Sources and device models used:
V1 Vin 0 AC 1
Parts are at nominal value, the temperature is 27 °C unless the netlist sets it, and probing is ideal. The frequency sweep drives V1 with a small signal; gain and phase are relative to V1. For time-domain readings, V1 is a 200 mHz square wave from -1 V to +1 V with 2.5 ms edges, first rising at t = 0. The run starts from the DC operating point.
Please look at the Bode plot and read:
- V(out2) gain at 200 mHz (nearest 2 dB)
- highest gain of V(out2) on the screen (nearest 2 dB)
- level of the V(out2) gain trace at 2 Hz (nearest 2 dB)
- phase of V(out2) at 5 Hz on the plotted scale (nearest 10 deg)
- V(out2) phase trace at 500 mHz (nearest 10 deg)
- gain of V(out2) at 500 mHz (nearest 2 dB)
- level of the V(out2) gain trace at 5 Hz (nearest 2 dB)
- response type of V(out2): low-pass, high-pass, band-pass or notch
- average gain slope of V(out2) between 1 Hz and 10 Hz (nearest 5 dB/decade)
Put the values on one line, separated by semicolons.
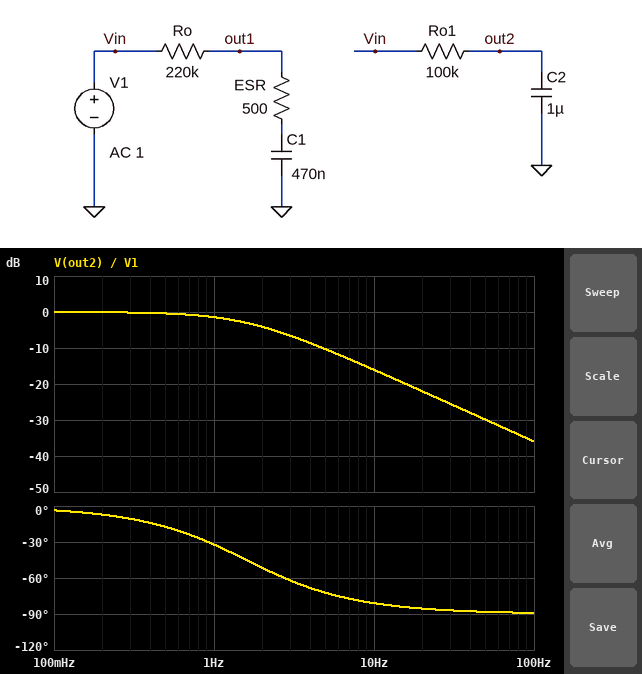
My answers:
0 dB; 0 dB; -4 dB; -70 deg; -20 deg; 0 dB; -10 dB; low-pass; -15 dB/decade
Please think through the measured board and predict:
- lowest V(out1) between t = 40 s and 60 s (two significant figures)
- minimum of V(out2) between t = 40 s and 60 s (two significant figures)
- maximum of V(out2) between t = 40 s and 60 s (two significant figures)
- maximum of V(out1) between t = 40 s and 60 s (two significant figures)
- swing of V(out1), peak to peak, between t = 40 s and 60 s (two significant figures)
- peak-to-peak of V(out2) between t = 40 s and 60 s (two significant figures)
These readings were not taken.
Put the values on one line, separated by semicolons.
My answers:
-1.0 V; -1.0 V; 1.0 V; 1.0 V; 2.0 V; 2.0 V
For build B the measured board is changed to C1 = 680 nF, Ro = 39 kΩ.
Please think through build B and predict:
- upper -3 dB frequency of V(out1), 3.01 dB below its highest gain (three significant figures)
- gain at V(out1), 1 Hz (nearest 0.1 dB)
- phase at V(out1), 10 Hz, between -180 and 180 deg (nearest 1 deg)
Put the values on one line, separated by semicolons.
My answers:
5.93 Hz; -0.1 dB; -58 deg
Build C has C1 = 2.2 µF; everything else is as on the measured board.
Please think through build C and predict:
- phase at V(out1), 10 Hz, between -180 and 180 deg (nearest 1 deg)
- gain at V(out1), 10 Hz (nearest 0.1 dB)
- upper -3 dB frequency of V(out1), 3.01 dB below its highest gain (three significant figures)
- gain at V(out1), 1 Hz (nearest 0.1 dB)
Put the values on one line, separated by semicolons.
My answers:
-84 deg; -29.7 dB; 328 mHz; -10.1 dB
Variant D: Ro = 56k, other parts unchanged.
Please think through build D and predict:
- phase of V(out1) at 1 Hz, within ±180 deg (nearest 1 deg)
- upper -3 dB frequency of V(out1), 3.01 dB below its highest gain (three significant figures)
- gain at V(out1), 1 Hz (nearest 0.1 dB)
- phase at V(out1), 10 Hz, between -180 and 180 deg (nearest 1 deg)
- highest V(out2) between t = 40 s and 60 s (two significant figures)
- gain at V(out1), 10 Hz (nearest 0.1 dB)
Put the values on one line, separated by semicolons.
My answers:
-9 deg; 5.99 Hz; -0.1 dB; -58 deg; 1.0 V; -5.8 dB
